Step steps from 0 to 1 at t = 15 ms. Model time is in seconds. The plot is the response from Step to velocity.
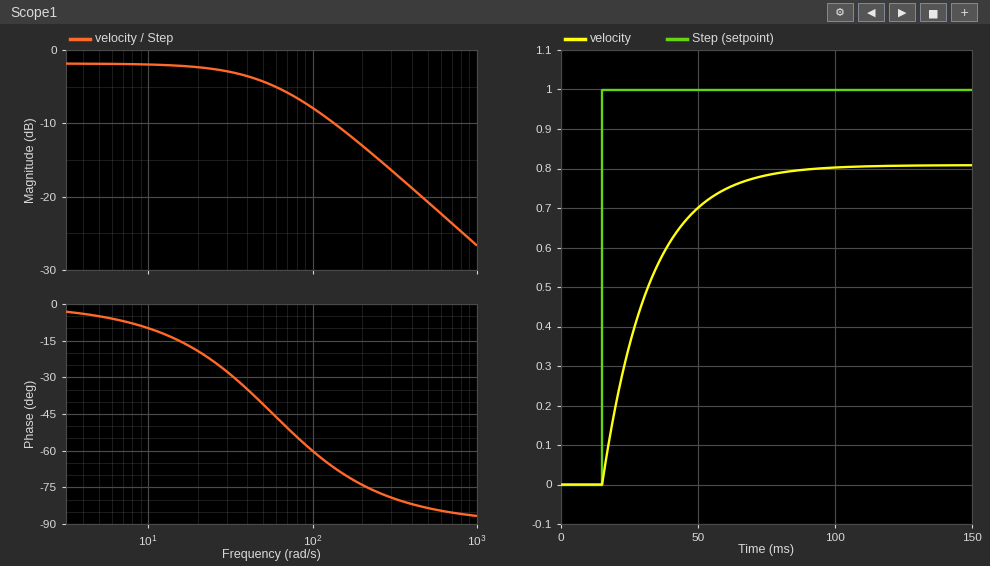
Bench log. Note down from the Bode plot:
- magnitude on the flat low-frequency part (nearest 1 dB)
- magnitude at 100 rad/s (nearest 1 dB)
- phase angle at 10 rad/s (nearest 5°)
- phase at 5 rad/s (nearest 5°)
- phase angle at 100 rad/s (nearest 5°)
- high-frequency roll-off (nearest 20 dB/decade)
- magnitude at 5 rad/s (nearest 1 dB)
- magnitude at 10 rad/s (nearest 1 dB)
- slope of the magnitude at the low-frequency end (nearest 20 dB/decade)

-2 dB
-8 dB
-10°
-5°
-60°
-20 dB/decade
-2 dB
-2 dB
0 dB/decade
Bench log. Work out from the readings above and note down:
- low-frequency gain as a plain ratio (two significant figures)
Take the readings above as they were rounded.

0.79
